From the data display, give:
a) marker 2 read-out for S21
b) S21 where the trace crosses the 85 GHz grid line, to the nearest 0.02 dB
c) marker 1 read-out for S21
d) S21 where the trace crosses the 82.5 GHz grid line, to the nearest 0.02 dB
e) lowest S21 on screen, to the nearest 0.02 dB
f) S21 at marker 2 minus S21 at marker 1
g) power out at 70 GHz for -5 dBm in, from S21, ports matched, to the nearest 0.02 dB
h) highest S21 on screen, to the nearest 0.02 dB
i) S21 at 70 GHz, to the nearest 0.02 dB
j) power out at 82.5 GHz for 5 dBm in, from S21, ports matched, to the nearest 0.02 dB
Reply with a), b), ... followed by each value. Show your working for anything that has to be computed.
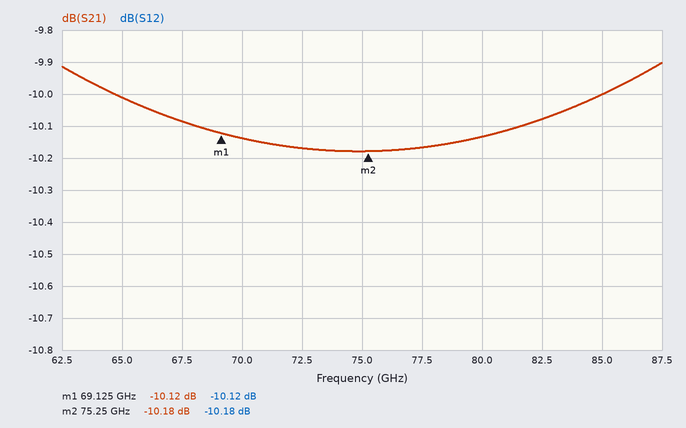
a) -10.18 dB
b) -10.00 dB
c) -10.12 dB
d) -10.08 dB
e) -10.18 dB
f) -10.18 − (-10.12) = -0.06 dB
g) -5 dBm + (-10.14 dB) = -15.14 dBm
h) -9.90 dB
i) -10.14 dB
j) 5 dBm + (-10.08 dB) = -5.08 dBm
